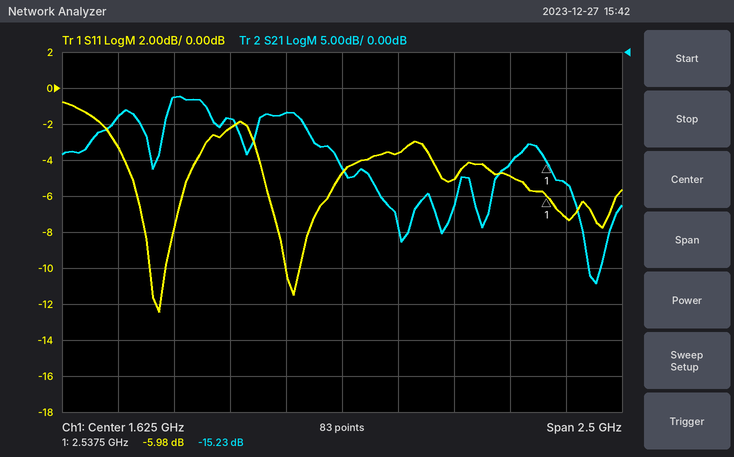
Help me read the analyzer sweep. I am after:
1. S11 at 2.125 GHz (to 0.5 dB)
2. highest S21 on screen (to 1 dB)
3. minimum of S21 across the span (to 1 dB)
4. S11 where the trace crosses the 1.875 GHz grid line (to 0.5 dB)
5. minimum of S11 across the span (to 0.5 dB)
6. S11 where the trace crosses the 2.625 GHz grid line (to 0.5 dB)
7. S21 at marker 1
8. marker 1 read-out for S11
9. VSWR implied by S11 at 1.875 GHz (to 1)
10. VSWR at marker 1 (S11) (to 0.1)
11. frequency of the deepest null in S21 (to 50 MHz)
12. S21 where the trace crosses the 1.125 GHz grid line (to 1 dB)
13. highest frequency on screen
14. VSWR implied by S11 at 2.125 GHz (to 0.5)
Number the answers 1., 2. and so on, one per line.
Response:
1. -5.0 dB
2. -6 dB
3. -32 dB
4. -3.5 dB
5. -12.5 dB
6. -7.0 dB
7. -15.23 dB
8. -5.98 dB
9. 5
10. 3.0
11. 2.75 GHz
12. -9 dB
13. 2.875 GHz
14. 3.5
